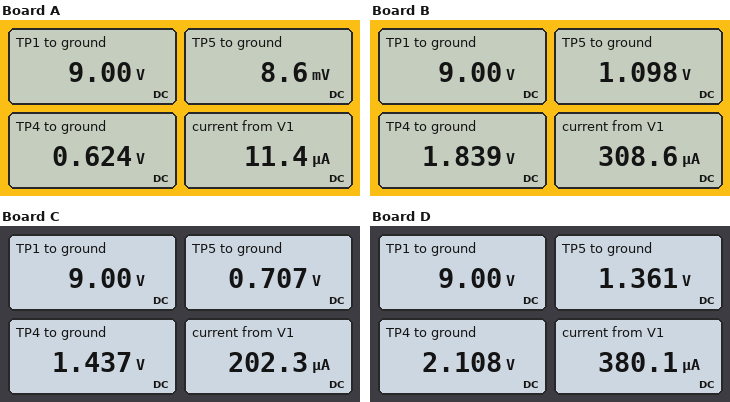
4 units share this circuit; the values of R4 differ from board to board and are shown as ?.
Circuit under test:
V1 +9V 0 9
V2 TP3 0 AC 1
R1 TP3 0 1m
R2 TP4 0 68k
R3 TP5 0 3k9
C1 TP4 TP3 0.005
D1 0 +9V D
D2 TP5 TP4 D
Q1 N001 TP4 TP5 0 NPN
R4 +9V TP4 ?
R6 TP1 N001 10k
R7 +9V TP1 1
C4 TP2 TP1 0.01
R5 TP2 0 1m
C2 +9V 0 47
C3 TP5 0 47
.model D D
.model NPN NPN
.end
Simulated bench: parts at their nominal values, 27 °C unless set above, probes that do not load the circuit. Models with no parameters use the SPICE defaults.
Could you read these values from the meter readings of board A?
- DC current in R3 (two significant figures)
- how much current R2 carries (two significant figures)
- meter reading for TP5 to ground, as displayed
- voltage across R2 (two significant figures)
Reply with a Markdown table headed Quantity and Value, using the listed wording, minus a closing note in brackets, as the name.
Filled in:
| Quantity | Value |
|---|---|
| DC current in R3 | 2.2 µA |
| how much current R2 carries | 9.2 µA |
| meter reading for TP5 to ground, as displayed | 8.6 mV |
| voltage across R2 | 620 mV |
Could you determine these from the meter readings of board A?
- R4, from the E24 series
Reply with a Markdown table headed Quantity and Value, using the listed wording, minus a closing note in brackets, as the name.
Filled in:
| Quantity | Value |
|---|---|
| R4, from the E24 series | 910 kΩ |
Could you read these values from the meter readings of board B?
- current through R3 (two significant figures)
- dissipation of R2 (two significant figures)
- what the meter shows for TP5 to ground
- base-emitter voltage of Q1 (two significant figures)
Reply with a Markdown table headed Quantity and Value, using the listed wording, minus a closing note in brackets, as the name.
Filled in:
| Quantity | Value |
|---|---|
| current through R3 | 280 µA |
| dissipation of R2 | 50 µW |
| what the meter shows for TP5 to ground | 1.098 V |
| base-emitter voltage of Q1 | 740 mV |
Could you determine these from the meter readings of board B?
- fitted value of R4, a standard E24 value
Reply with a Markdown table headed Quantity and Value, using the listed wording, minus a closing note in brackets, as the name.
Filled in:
| Quantity | Value |
|---|---|
| fitted value of R4, a standard E24 value | 240 kΩ |
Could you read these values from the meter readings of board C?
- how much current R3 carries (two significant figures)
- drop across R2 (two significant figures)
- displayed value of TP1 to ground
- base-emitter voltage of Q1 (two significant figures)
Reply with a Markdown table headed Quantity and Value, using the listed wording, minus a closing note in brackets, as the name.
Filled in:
| Quantity | Value |
|---|---|
| how much current R3 carries | 180 µA |
| drop across R2 | 1.4 V |
| displayed value of TP1 to ground | 9.00 V |
| base-emitter voltage of Q1 | 730 mV |
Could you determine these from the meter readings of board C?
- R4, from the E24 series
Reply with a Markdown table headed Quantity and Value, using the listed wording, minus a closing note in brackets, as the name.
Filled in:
| Quantity | Value |
|---|---|
| R4, from the E24 series | 330 kΩ |
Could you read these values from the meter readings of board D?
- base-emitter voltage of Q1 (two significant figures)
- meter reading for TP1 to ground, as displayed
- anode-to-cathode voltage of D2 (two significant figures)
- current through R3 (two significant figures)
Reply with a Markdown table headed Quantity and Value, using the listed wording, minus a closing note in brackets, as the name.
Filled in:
| Quantity | Value |
|---|---|
| base-emitter voltage of Q1 | 750 mV |
| meter reading for TP1 to ground, as displayed | 9.00 V |
| anode-to-cathode voltage of D2 | -750 mV |
| current through R3 | 350 µA |
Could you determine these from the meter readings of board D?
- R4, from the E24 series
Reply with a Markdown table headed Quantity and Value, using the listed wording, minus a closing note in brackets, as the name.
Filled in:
| Quantity | Value |
|---|---|
| R4, from the E24 series | 200 kΩ |
